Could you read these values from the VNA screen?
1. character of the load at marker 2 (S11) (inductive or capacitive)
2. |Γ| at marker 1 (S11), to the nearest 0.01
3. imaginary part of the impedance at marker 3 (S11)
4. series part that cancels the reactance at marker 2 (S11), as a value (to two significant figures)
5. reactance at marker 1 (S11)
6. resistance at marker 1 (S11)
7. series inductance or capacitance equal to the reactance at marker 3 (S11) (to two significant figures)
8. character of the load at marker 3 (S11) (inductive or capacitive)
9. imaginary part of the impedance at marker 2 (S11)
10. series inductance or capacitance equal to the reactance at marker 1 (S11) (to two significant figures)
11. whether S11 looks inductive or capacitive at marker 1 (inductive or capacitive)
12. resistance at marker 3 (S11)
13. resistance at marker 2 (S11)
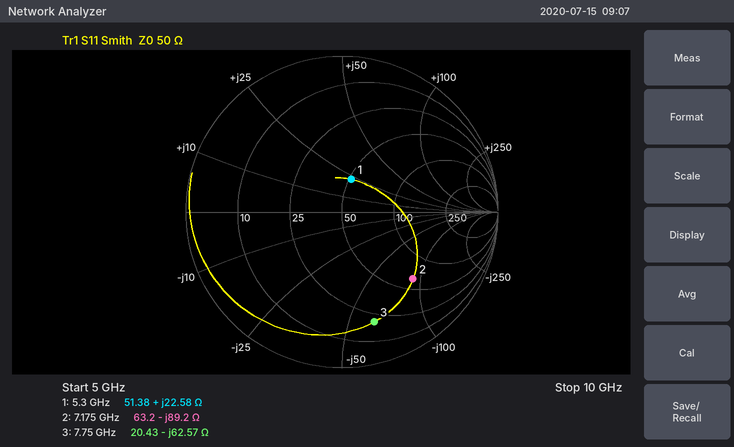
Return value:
capacitive
0.22
-62.57 Ω
2.0 nH
+22.58 Ω
51.38 Ω
330 fF
capacitive
-89.2 Ω
680 pH
inductive
20.43 Ω
63.2 Ω
